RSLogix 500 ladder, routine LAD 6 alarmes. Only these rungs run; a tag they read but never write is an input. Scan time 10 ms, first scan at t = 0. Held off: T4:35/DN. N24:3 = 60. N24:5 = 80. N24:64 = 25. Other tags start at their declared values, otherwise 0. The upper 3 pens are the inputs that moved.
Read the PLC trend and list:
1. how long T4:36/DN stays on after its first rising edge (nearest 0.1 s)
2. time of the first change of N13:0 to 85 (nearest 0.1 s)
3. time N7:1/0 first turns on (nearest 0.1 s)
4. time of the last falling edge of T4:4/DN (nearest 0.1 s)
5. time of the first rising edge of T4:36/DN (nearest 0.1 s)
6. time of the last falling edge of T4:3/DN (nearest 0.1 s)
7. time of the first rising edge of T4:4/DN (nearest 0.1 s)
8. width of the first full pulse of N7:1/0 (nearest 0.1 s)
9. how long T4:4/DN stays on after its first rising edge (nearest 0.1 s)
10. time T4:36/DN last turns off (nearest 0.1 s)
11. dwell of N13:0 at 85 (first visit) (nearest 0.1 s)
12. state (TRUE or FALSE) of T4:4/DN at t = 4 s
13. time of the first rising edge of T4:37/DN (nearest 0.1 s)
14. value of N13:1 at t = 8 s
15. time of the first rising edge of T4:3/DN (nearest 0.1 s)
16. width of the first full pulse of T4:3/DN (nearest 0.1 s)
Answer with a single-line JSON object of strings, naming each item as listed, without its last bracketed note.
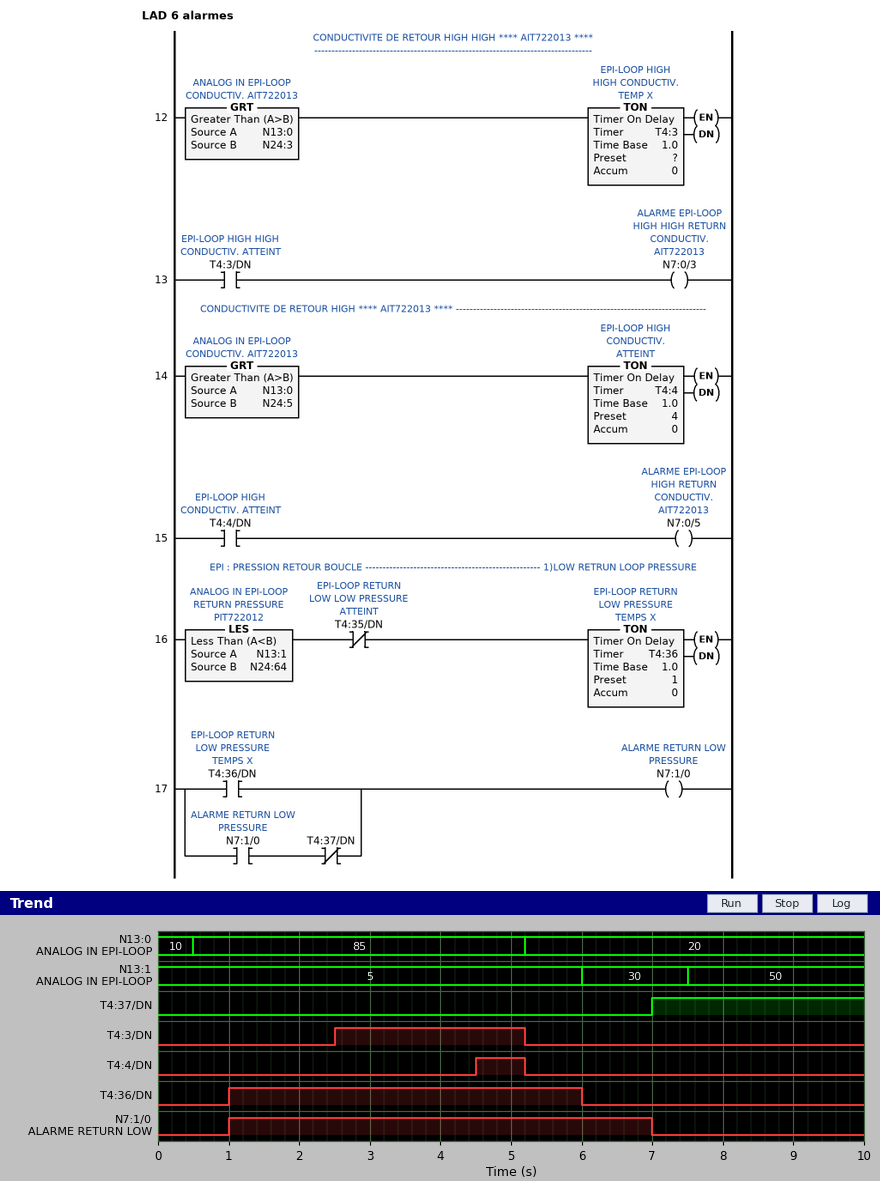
{"how long T4:36/DN stays on after its first rising edge": "5.0 s", "time of the first change of N13:0 to 85": "0.5 s", "time N7:1/0 first turns on": "1.0 s", "time of the last falling edge of T4:4/DN": "5.2 s", "time of the first rising edge of T4:36/DN": "1.0 s", "time of the last falling edge of T4:3/DN": "5.2 s", "time of the first rising edge of T4:4/DN": "4.5 s", "width of the first full pulse of N7:1/0": "6.0 s", "how long T4:4/DN stays on after its first rising edge": "0.7 s", "time T4:36/DN last turns off": "6.0 s", "dwell of N13:0 at 85 (first visit)": "4.7 s", "state (TRUE or FALSE) of T4:4/DN at t = 4 s": "FALSE", "time of the first rising edge of T4:37/DN": "7.0 s", "value of N13:1 at t = 8 s": "50", "time of the first rising edge of T4:3/DN": "2.5 s", "width of the first full pulse of T4:3/DN": "2.7 s"}
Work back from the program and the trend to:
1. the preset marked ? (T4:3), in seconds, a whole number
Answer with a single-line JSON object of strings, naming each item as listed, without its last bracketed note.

{"the preset marked ? (T4:3), in seconds, a whole number": "2 s"}
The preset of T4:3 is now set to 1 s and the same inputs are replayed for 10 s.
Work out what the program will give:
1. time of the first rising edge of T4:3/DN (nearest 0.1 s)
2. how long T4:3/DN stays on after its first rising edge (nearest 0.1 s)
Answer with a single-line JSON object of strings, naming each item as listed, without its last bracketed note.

{"time of the first rising edge of T4:3/DN": "1.5 s", "how long T4:3/DN stays on after its first rising edge": "3.7 s"}
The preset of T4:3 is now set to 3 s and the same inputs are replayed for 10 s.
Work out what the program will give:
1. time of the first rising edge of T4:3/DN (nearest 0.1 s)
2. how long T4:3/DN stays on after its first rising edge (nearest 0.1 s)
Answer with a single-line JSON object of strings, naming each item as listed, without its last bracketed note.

{"time of the first rising edge of T4:3/DN": "3.5 s", "how long T4:3/DN stays on after its first rising edge": "1.7 s"}
